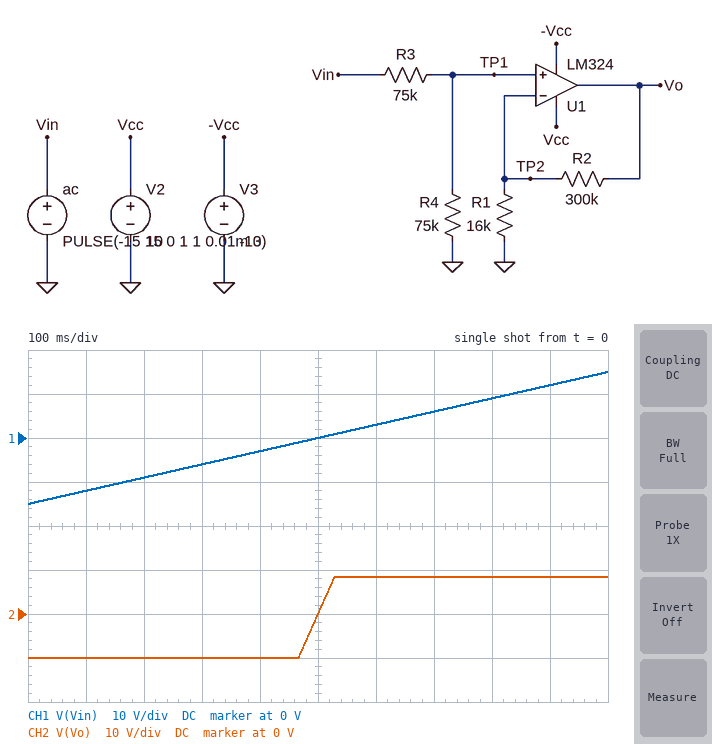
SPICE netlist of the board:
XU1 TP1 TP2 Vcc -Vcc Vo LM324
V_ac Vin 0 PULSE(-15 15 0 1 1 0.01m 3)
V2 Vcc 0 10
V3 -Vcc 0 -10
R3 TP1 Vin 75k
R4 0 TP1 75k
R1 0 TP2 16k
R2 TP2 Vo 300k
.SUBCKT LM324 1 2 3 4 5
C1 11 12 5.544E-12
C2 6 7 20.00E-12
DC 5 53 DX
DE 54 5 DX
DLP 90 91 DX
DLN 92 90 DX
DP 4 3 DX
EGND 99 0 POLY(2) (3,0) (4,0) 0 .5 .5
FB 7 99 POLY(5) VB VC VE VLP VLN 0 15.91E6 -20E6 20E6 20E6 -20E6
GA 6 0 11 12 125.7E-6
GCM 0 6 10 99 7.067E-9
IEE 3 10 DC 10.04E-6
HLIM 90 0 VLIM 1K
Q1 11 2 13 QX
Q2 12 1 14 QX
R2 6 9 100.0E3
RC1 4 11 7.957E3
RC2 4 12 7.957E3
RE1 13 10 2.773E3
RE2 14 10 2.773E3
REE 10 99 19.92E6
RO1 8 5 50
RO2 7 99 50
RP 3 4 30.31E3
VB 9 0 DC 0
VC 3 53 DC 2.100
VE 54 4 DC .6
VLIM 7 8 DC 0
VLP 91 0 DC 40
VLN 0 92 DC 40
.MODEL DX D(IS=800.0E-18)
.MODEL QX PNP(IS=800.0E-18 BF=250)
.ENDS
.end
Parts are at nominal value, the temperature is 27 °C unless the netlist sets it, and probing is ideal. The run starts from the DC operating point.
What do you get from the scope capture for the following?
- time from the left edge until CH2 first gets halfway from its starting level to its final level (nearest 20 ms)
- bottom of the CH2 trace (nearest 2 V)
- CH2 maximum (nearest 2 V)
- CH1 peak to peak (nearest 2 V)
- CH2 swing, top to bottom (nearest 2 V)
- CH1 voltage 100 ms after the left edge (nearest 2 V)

500 ms
-10 V
8 V
30 V
18 V
-12 V
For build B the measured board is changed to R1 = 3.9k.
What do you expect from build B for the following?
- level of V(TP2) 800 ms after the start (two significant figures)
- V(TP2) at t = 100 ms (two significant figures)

110 mV
-130 mV
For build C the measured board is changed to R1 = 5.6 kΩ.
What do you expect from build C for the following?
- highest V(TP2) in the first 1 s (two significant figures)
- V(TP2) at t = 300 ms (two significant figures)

160 mV
-180 mV
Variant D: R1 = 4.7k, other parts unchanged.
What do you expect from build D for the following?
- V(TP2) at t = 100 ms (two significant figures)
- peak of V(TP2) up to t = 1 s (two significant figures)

-150 mV
130 mV
